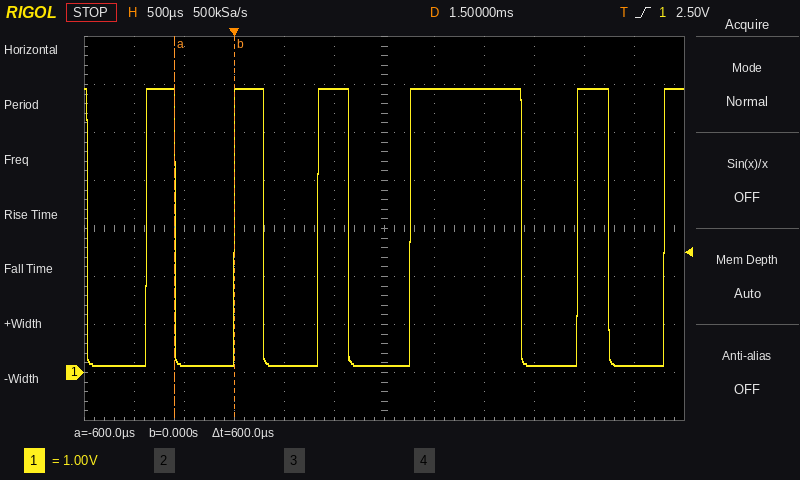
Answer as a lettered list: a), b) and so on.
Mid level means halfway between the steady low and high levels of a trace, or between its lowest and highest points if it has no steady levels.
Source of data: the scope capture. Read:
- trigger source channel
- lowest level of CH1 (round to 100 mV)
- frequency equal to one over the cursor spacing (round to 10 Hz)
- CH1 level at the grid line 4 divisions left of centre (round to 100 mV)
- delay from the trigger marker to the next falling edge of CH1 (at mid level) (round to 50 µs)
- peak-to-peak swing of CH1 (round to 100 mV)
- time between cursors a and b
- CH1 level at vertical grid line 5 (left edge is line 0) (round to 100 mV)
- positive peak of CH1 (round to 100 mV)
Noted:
a) CH1
b) 100 mV
c) 1.67 kHz
d) 100 mV
e) 300 µs
f) 5.8 V
g) 600 µs
h) 5.9 V
i) 5.9 V
